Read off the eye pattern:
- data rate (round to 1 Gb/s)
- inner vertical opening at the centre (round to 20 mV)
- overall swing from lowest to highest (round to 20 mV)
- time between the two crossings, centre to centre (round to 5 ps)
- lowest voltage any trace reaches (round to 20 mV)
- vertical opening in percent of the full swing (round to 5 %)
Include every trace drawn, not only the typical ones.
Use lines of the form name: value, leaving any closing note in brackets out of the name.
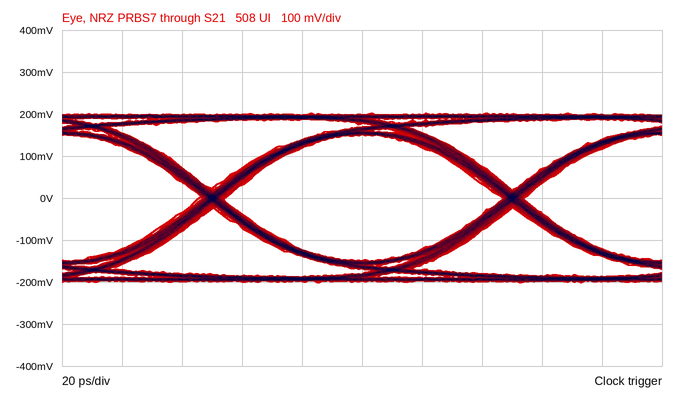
data rate: 10 Gb/s
inner vertical opening at the centre: 300 mV
overall swing from lowest to highest: 400 mV
time between the two crossings, centre to centre: 100 ps
lowest voltage any trace reaches: -200 mV
vertical opening in percent of the full swing: 75 %
